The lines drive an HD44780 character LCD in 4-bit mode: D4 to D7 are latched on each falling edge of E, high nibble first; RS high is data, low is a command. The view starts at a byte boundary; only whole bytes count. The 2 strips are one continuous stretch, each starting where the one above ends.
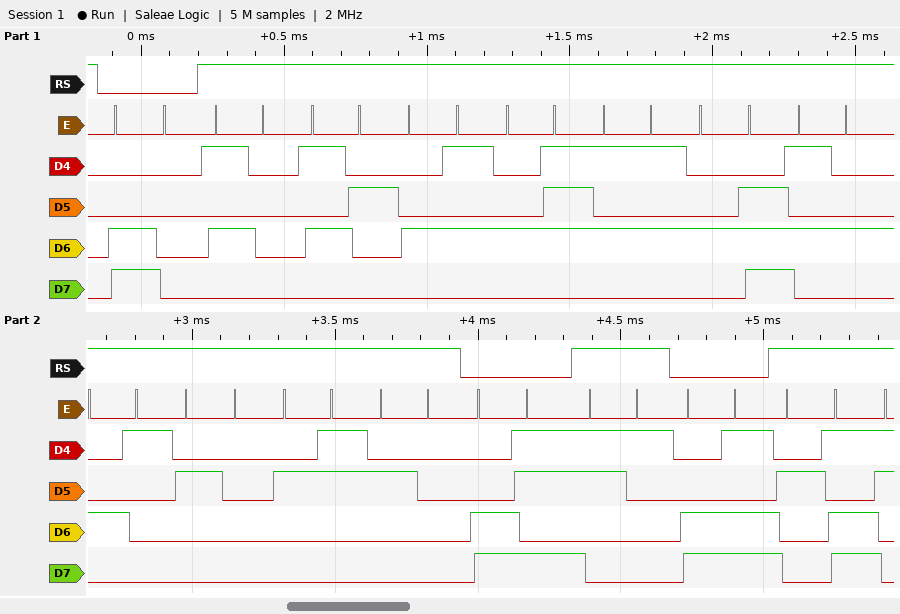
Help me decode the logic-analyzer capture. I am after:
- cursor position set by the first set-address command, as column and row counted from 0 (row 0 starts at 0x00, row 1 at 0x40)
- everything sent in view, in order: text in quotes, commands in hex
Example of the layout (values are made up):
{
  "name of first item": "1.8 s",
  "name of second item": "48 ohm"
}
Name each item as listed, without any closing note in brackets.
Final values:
{
  "cursor position set by the first set-address command, as column and row counted from 0": "column 0, row 1",
  "everything sent in view, in order: text in quotes, commands in hex": "0xC0 \"PREGUNTA # \" 0xCB \"1\" 0xCD \"-\""
}
